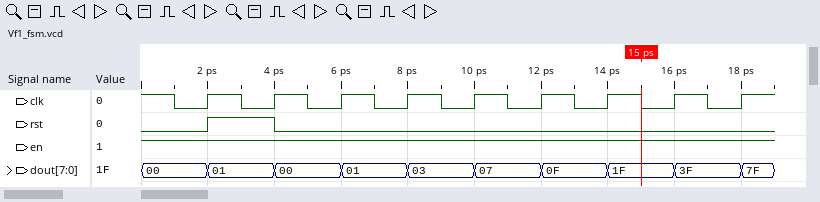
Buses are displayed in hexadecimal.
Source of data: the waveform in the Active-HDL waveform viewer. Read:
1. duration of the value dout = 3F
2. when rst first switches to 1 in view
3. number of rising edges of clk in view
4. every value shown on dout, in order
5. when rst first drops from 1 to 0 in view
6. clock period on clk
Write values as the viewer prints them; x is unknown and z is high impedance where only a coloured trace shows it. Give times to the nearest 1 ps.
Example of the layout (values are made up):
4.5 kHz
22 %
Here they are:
2 ps
2 ps
9
00, 01, 00, 01, 03, 07, 0F, 1F, 3F, 7F
4 ps
2 ps
